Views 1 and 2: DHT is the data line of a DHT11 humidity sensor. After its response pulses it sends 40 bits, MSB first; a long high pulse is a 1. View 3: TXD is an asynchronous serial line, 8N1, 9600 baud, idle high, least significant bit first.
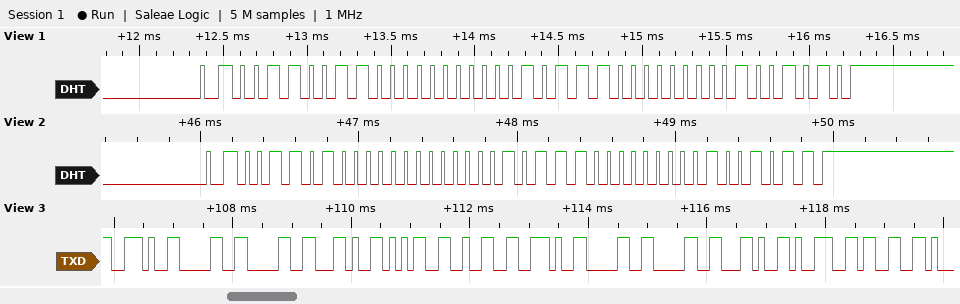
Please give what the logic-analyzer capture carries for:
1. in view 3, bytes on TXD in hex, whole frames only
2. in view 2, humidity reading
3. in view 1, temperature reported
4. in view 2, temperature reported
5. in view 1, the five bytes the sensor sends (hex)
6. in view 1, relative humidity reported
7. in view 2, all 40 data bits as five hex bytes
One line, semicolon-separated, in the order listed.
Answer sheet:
0x2E 0x30 0x30 0x2C 0x35 0x32 0x2E 0x30 0x30 0x2C 0x39 0x33; 52 %; 23.0 °C; 23.0 °C; 33 00 17 00 4A; 51 %; 34 00 17 00 4B
